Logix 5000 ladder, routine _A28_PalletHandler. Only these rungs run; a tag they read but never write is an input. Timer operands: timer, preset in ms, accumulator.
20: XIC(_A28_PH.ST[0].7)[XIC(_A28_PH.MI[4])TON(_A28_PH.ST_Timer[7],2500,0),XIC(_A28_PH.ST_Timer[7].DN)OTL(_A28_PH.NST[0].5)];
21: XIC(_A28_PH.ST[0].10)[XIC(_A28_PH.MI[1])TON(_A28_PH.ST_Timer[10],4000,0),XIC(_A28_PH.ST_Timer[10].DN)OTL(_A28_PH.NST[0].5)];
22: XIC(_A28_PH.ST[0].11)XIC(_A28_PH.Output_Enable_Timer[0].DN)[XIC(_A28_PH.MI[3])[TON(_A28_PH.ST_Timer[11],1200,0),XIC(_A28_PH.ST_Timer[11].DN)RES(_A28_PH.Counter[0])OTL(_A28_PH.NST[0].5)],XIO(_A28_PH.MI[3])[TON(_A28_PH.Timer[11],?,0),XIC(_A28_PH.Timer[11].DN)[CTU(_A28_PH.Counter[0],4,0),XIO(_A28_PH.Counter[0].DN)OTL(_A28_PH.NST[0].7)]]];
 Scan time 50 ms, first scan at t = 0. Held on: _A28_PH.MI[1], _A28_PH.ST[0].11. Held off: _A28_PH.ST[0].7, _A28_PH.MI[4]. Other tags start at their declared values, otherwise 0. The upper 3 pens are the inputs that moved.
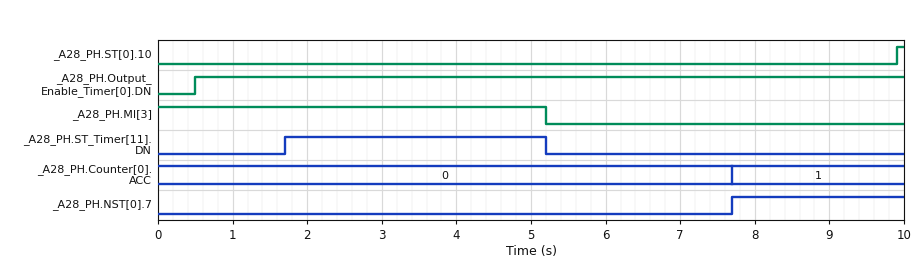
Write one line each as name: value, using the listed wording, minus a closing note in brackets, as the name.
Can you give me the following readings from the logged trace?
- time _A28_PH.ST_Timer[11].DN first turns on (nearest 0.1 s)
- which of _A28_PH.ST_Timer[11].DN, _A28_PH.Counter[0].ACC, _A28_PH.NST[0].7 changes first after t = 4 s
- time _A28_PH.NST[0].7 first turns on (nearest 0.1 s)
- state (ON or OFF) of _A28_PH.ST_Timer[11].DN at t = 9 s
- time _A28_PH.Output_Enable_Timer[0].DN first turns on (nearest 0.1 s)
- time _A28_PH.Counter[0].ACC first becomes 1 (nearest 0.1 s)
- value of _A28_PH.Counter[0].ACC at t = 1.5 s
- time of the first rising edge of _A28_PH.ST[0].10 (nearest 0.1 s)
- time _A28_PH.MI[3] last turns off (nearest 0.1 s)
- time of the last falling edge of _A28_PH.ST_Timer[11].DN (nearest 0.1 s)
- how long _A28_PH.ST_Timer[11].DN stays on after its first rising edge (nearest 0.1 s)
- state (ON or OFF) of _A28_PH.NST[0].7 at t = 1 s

time _A28_PH.ST_Timer[11].DN first turns on: 1.7 s
which of _A28_PH.ST_Timer[11].DN, _A28_PH.Counter[0].ACC, _A28_PH.NST[0].7 changes first after t = 4 s: _A28_PH.ST_Timer[11].DN
time _A28_PH.NST[0].7 first turns on: 7.7 s
state (ON or OFF) of _A28_PH.ST_Timer[11].DN at t = 9 s: OFF
time _A28_PH.Output_Enable_Timer[0].DN first turns on: 0.5 s
time _A28_PH.Counter[0].ACC first becomes 1: 7.7 s
value of _A28_PH.Counter[0].ACC at t = 1.5 s: 0
time of the first rising edge of _A28_PH.ST[0].10: 9.9 s
time _A28_PH.MI[3] last turns off: 5.2 s
time of the last falling edge of _A28_PH.ST_Timer[11].DN: 5.2 s
how long _A28_PH.ST_Timer[11].DN stays on after its first rising edge: 3.5 s
state (ON or OFF) of _A28_PH.NST[0].7 at t = 1 s: OFF
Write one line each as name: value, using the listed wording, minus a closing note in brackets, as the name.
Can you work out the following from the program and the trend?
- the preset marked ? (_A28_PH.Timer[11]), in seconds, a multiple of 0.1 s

the preset marked ? (_A28_PH.Timer[11]), in seconds, a multiple of 0.1 s: 2.5 s
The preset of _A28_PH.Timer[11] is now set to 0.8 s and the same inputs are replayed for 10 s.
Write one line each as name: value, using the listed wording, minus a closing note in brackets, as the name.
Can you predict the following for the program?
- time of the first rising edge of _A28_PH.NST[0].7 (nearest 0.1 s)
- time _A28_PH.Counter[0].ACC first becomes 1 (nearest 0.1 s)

time of the first rising edge of _A28_PH.NST[0].7: 6.0 s
time _A28_PH.Counter[0].ACC first becomes 1: 6.0 s
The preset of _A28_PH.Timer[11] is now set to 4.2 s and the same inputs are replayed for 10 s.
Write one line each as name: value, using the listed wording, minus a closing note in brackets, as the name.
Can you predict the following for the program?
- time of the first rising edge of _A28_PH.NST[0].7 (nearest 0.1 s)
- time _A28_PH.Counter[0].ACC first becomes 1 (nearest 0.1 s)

time of the first rising edge of _A28_PH.NST[0].7: 9.4 s
time _A28_PH.Counter[0].ACC first becomes 1: 9.4 s
